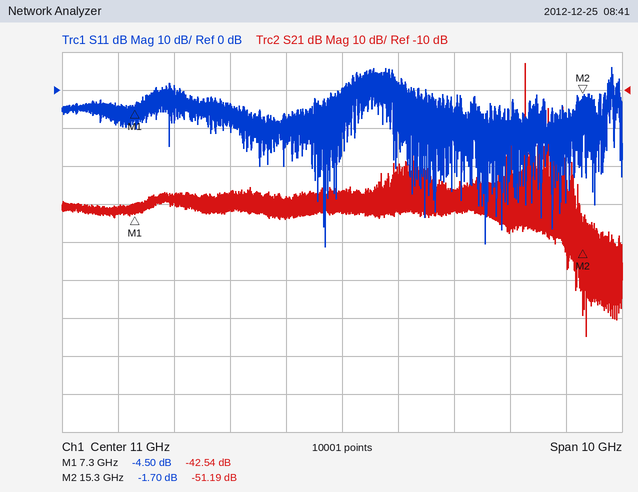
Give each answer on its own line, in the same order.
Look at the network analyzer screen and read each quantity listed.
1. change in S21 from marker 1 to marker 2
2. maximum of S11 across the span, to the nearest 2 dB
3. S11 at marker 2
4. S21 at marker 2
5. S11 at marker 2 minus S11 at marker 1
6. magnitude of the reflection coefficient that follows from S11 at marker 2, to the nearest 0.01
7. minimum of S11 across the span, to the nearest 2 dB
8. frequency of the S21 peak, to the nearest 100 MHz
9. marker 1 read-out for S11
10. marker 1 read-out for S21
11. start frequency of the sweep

-8.65 dB
6 dB
-1.70 dB
-51.19 dB
2.80 dB
0.82
-42 dB
14.3 GHz
-4.50 dB
-42.54 dB
6 GHz
